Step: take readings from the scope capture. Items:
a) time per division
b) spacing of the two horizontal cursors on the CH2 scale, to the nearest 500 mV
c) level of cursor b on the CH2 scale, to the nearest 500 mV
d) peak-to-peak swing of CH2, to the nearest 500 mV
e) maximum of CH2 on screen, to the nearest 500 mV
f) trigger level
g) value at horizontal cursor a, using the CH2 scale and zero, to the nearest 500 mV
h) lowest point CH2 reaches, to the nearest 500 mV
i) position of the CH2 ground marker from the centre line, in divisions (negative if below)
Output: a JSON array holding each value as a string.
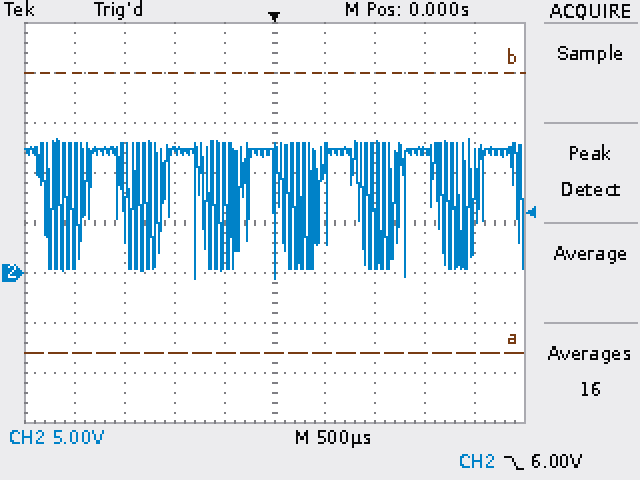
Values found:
["500 µs", "28.0 V", "20.0 V", "14.0 V", "13.5 V", "6.00 V", "-8.0 V", "-500 mV", "-1.0 div"]
